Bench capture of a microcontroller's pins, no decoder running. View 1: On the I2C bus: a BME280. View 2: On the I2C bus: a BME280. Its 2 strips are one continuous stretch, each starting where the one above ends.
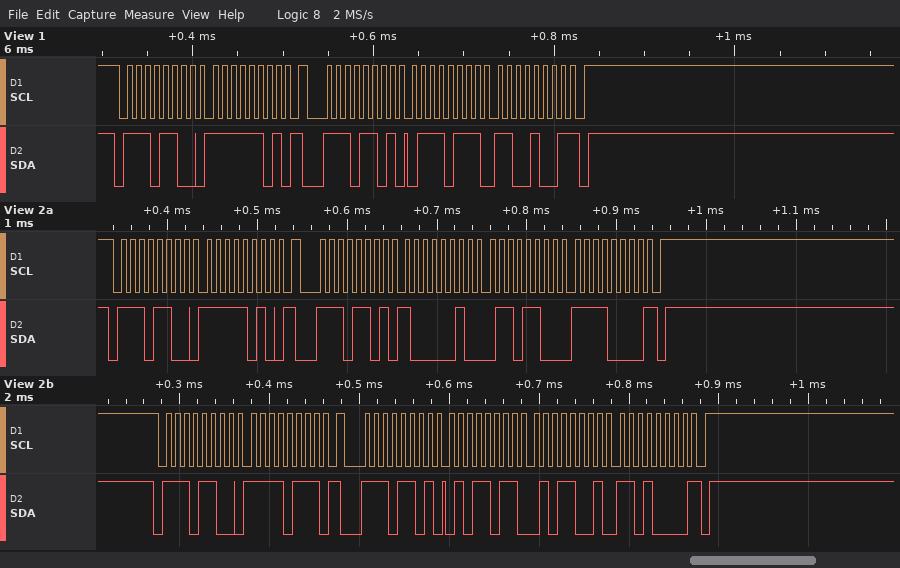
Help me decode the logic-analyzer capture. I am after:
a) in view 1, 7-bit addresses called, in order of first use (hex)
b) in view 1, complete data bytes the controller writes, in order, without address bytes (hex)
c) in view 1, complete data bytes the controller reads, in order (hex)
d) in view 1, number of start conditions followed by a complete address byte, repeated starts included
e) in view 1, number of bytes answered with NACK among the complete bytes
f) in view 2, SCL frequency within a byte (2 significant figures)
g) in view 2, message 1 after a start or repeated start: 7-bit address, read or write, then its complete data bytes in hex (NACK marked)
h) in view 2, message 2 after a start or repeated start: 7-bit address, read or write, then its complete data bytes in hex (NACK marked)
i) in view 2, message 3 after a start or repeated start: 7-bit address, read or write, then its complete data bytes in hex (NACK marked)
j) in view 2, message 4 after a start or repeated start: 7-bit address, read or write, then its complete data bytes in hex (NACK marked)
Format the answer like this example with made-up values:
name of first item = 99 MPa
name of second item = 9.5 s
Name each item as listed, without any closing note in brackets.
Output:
in view 1, 7-bit addresses called, in order of first use = 0x76
in view 1, complete data bytes the controller writes, in order, without address bytes = FD
in view 1, complete data bytes the controller reads, in order = 77 C9
in view 1, number of start conditions followed by a complete address byte, repeated starts included = 2
in view 1, number of bytes answered with NACK among the complete bytes = 1
in view 2, SCL frequency within a byte = 100 kHz
in view 2, message 1 after a start or repeated start: 7-bit address, read or write, then its complete data bytes in hex = 0x76 write: FA
in view 2, message 2 after a start or repeated start: 7-bit address, read or write, then its complete data bytes in hex = 0x76 read: 82 6C F0 NACK
in view 2, message 3 after a start or repeated start: 7-bit address, read or write, then its complete data bytes in hex = 0x76 write: F7
in view 2, message 4 after a start or repeated start: 7-bit address, read or write, then its complete data bytes in hex = 0x76 read: 5B 59 D0 NACK
